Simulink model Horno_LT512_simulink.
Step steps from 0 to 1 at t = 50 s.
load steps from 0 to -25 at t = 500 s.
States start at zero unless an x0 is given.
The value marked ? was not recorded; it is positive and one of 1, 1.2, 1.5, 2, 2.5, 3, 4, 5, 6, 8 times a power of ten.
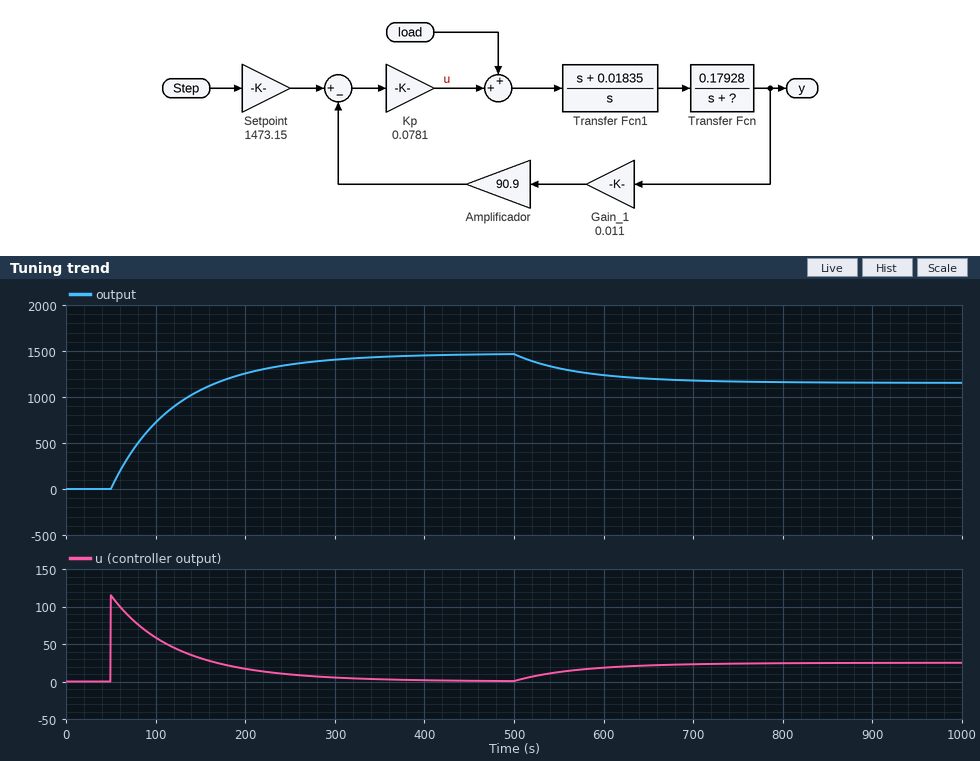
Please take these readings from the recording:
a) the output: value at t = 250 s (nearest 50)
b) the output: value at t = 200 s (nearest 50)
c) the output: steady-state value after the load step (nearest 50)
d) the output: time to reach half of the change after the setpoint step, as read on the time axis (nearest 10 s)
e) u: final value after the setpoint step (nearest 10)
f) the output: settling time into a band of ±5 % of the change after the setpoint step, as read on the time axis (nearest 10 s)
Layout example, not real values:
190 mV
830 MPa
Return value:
1350
1250
1150
100 s
0
290 s
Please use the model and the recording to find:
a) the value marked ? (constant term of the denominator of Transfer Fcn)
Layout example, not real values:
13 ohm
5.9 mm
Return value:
0.02
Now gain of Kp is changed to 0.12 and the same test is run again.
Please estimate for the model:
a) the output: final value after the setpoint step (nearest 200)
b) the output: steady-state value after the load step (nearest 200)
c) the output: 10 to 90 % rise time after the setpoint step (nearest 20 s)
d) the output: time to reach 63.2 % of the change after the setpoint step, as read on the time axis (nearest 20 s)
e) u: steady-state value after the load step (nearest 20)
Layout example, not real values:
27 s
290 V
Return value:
1400
1200
120 s
100 s
20
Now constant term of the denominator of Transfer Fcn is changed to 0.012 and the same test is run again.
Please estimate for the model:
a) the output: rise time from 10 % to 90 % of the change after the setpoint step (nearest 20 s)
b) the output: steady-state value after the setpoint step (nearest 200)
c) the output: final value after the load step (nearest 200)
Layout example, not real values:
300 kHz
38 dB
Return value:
100 s
1400
1200
